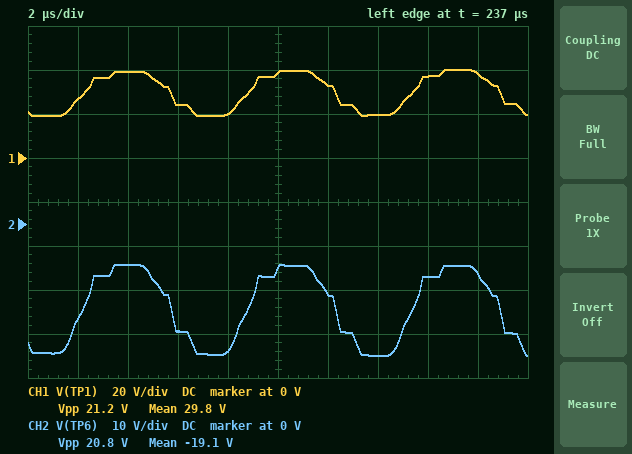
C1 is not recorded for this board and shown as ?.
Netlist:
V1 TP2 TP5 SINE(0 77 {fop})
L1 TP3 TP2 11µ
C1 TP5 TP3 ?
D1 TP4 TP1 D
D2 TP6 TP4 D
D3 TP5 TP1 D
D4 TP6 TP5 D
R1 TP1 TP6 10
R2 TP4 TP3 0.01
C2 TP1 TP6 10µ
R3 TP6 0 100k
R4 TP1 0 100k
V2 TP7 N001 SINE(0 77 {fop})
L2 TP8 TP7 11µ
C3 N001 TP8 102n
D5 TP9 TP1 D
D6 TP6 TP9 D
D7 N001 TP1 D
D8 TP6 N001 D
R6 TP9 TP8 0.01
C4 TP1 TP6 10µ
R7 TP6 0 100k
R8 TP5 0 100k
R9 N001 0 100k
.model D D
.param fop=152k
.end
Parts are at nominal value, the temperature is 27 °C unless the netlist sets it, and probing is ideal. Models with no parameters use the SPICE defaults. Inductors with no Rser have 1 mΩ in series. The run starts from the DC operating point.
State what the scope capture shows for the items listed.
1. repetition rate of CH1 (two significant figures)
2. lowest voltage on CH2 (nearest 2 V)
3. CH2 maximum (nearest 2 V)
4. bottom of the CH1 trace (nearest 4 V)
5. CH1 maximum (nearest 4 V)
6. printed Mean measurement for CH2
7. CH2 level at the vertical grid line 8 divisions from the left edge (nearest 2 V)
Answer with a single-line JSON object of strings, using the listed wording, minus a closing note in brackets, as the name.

{"repetition rate of CH1": "150 kHz", "lowest voltage on CH2": "-30 V", "CH2 maximum": "-10 V", "bottom of the CH1 trace": "20 V", "CH1 maximum": "40 V", "printed Mean measurement for CH2": "-19.1 V", "CH2 level at the vertical grid line 8 divisions from the left edge": "-12 V"}
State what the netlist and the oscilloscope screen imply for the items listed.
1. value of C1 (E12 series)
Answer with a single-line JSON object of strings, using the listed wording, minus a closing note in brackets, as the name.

{"value of C1": "180 nF"}
